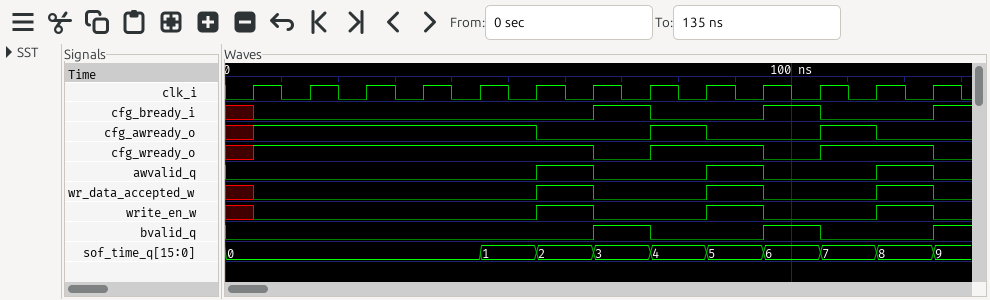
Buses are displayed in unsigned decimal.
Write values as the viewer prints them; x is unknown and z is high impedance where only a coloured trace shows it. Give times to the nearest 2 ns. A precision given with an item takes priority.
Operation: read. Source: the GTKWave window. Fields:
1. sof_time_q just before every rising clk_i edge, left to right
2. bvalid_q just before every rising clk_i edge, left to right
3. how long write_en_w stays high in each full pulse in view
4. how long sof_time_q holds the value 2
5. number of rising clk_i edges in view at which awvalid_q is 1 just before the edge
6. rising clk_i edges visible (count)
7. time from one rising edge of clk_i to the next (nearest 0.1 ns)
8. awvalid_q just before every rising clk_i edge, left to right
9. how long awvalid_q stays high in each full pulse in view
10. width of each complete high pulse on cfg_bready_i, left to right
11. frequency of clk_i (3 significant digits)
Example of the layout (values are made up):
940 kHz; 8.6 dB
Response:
0, 0, 0, 0, 0, 1, 2, 3, 4, 5, 6, 7, 8; 0 0 0 0 0 0 0 1 0 0 1 0 0; 10 ns, 10 ns, 10 ns; 10 ns; 3; 13; 10 ns; 0 0 0 0 0 0 1 0 0 1 0 0 1; 10 ns, 10 ns, 10 ns; 10 ns, 10 ns; 100 MHz
